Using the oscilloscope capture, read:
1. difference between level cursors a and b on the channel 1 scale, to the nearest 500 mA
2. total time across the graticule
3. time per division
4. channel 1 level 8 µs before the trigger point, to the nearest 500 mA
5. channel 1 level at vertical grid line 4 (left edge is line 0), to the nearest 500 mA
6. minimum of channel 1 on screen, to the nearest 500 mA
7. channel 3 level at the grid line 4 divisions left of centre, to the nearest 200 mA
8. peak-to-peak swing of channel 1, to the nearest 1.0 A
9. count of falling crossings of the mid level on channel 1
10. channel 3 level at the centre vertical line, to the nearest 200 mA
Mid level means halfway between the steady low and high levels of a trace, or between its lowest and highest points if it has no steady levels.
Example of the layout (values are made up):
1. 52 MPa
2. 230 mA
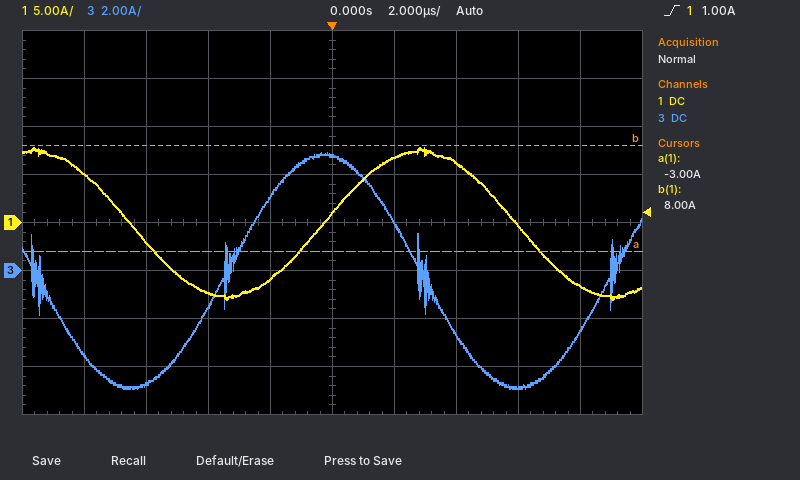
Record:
1. 11.0 A
2. 20 µs
3. 2 µs
4. 5.0 A
5. -6.0 A
6. -8.0 A
7. -3.6 A
8. 16.0 A
9. 2
10. 4.8 A
